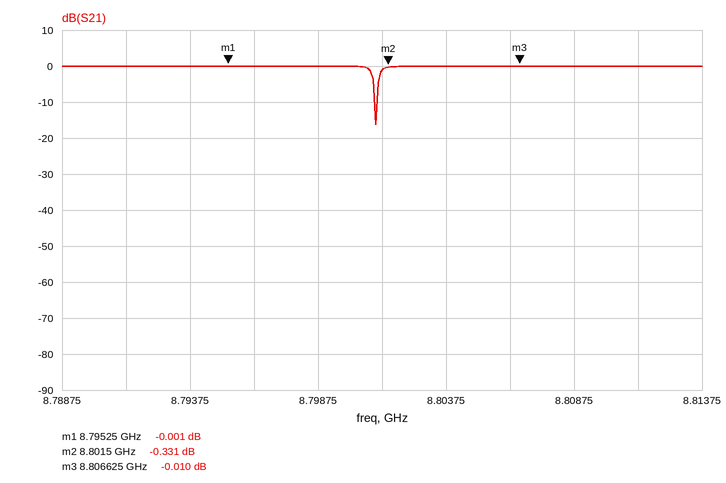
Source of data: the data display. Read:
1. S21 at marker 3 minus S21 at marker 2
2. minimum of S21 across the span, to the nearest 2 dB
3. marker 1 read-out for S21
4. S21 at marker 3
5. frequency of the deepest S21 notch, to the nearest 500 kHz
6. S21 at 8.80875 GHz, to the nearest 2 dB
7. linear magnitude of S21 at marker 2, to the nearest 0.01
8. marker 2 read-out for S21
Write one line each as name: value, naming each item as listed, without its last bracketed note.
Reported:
S21 at marker 3 minus S21 at marker 2: 0.321 dB
minimum of S21 across the span, to the nearest 2 dB: -16 dB
marker 1 read-out for S21: -0.001 dB
S21 at marker 3: -0.010 dB
frequency of the deepest S21 notch, to the nearest 500 kHz: 8.8010 GHz
S21 at 8.80875 GHz, to the nearest 2 dB: 0 dB
linear magnitude of S21 at marker 2, to the nearest 0.01: 0.96
marker 2 read-out for S21: -0.331 dB
